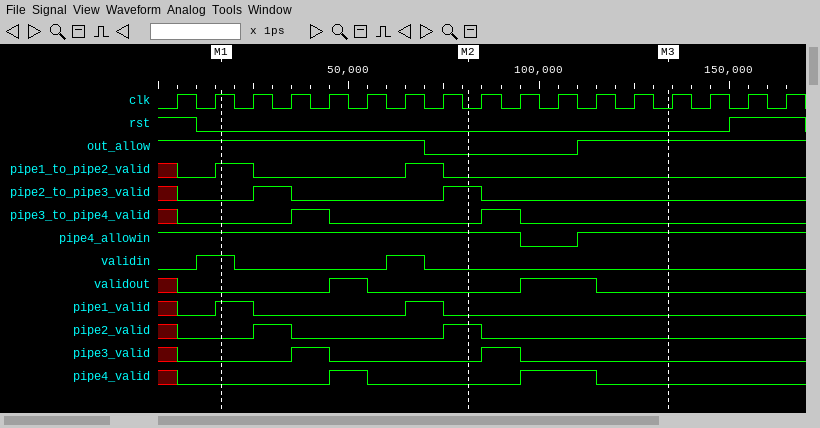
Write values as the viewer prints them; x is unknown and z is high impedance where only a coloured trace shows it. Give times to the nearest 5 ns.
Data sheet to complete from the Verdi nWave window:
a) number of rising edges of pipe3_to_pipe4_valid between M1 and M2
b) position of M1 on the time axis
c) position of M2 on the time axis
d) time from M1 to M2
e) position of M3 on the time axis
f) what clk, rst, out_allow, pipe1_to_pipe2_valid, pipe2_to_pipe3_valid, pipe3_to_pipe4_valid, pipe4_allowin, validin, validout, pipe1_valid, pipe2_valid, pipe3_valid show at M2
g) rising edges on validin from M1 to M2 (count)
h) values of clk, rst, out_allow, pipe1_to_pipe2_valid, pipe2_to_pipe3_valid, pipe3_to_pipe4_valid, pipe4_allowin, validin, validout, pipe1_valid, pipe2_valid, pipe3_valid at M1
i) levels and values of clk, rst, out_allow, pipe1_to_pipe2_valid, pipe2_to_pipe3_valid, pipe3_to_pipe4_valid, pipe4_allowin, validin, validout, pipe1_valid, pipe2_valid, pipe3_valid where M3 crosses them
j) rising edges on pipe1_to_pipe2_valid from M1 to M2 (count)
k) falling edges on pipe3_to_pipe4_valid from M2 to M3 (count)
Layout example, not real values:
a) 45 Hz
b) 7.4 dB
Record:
a) 1
b) 15 ns
c) 80 ns
d) 65 ns
e) 135 ns
f) clk=0, rst=0, out_allow=0, pipe1_to_pipe2_valid=0, pipe2_to_pipe3_valid=1, pipe3_to_pipe4_valid=0, pipe4_allowin=1, validin=0, validout=0, pipe1_valid=0, pipe2_valid=1, pipe3_valid=0
g) 1
h) clk=1, rst=0, out_allow=1, pipe1_to_pipe2_valid=1, pipe2_to_pipe3_valid=0, pipe3_to_pipe4_valid=0, pipe4_allowin=1, validin=1, validout=0, pipe1_valid=1, pipe2_valid=0, pipe3_valid=0
i) clk=0, rst=0, out_allow=1, pipe1_to_pipe2_valid=0, pipe2_to_pipe3_valid=0, pipe3_to_pipe4_valid=0, pipe4_allowin=1, validin=0, validout=0, pipe1_valid=0, pipe2_valid=0, pipe3_valid=0
j) 1
k) 1
